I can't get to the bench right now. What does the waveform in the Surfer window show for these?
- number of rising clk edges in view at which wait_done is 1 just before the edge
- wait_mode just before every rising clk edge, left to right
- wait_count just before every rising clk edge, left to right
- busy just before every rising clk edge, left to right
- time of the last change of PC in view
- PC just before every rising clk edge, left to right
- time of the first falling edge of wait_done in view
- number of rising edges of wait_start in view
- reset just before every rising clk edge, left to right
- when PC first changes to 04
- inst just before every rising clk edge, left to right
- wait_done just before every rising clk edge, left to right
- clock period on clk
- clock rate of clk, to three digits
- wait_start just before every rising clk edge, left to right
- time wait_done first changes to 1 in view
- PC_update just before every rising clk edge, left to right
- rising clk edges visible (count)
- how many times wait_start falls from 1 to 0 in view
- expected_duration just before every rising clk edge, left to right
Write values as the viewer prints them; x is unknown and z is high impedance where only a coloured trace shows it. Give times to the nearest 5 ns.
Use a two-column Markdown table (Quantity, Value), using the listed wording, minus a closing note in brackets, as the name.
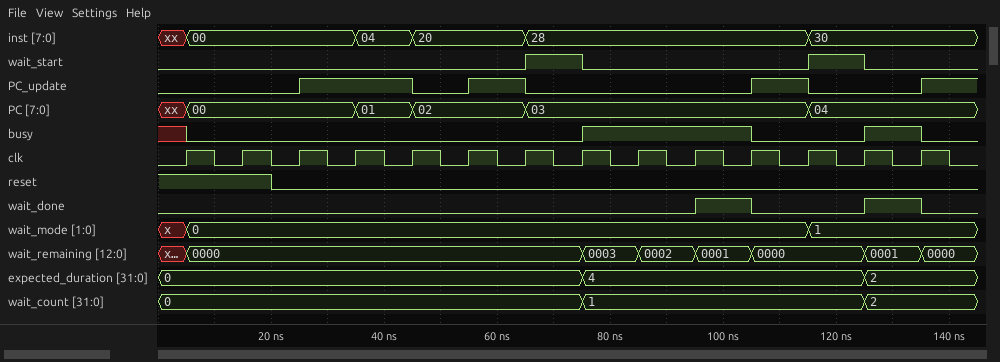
| Quantity | Value |
|---|---|
| number of rising clk edges in view at which wait_done is 1 just before the edge | 2 |
| wait_mode just before every rising clk edge, left to right | x, 0, 0, 0, 0, 0, 0, 0, 0, 0, 0, 0, 1, 1 |
| wait_count just before every rising clk edge, left to right | 0, 0, 0, 0, 0, 0, 0, 0, 1, 1, 1, 1, 1, 2 |
| busy just before every rising clk edge, left to right | x 0 0 0 0 0 0 0 1 1 1 0 0 1 |
| time of the last change of PC in view | 115 ns |
| PC just before every rising clk edge, left to right | xx, 00, 00, 00, 01, 02, 02, 03, 03, 03, 03, 03, 04, 04 |
| time of the first falling edge of wait_done in view | 105 ns |
| number of rising edges of wait_start in view | 2 |
| reset just before every rising clk edge, left to right | 1 1 0 0 0 0 0 0 0 0 0 0 0 0 |
| when PC first changes to 04 | 115 ns |
| inst just before every rising clk edge, left to right | xx, 00, 00, 00, 04, 20, 20, 28, 28, 28, 28, 28, 30, 30 |
| wait_done just before every rising clk edge, left to right | 0 0 0 0 0 0 0 0 0 0 1 0 0 1 |
| clock period on clk | 10 ns |
| clock rate of clk, to three digits | 100 MHz |
| wait_start just before every rising clk edge, left to right | 0 0 0 0 0 0 0 1 0 0 0 0 1 0 |
| time wait_done first changes to 1 in view | 95 ns |
| PC_update just before every rising clk edge, left to right | 0 0 0 1 1 0 1 0 0 0 0 1 0 0 |
| rising clk edges visible | 14 |
| how many times wait_start falls from 1 to 0 in view | 2 |
| expected_duration just before every rising clk edge, left to right | 0, 0, 0, 0, 0, 0, 0, 0, 4, 4, 4, 4, 4, 2 |
